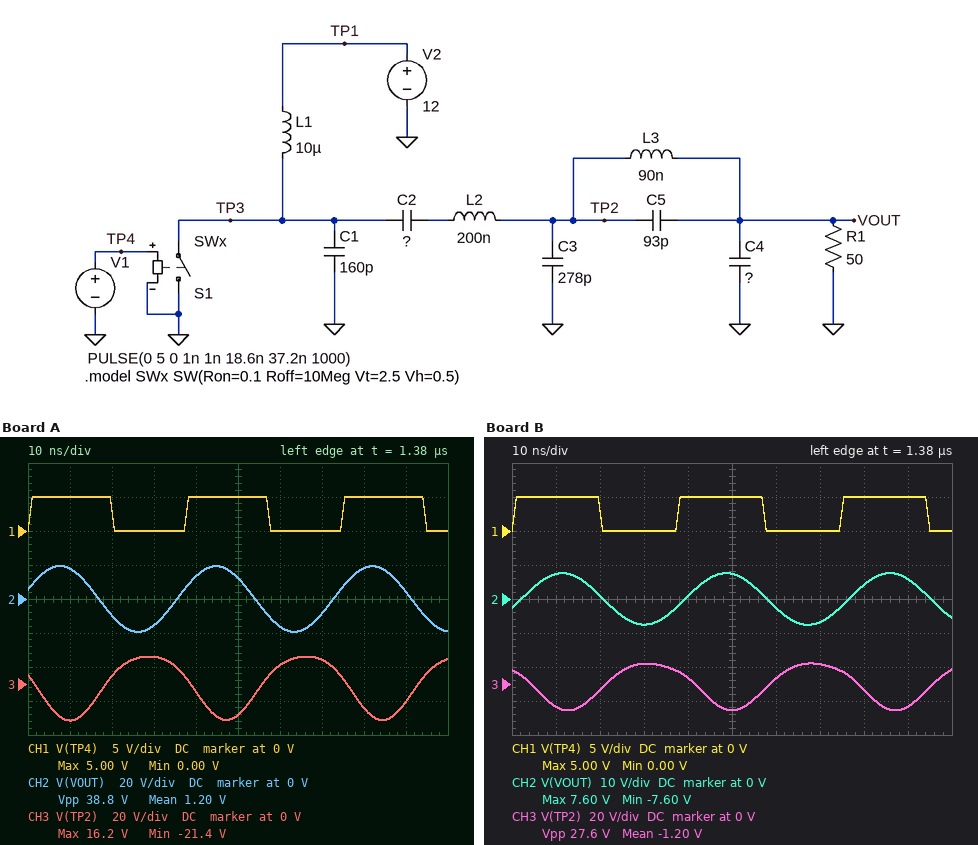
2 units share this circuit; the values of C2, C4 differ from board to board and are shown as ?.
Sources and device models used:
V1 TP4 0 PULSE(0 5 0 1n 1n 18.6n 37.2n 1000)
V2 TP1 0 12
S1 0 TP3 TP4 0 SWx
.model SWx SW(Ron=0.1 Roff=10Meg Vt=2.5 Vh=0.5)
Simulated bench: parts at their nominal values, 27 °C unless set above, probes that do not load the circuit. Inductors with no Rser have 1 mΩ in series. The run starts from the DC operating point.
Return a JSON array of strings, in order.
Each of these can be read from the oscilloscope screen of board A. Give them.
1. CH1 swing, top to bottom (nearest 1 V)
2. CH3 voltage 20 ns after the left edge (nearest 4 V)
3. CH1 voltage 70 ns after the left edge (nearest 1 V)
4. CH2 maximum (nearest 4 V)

["5 V", "4 V", "0 V", "20 V"]
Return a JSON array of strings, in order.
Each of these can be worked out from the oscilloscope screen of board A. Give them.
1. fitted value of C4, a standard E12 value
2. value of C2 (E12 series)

["560 pF", "180 pF"]
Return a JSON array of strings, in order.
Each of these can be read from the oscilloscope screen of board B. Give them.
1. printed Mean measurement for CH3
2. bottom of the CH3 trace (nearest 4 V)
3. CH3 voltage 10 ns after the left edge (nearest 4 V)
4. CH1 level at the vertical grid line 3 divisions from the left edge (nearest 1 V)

["-1.20 V", "-16 V", "-12 V", "0 V"]
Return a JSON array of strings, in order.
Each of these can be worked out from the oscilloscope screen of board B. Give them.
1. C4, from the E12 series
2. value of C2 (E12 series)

["820 pF", "270 pF"]
